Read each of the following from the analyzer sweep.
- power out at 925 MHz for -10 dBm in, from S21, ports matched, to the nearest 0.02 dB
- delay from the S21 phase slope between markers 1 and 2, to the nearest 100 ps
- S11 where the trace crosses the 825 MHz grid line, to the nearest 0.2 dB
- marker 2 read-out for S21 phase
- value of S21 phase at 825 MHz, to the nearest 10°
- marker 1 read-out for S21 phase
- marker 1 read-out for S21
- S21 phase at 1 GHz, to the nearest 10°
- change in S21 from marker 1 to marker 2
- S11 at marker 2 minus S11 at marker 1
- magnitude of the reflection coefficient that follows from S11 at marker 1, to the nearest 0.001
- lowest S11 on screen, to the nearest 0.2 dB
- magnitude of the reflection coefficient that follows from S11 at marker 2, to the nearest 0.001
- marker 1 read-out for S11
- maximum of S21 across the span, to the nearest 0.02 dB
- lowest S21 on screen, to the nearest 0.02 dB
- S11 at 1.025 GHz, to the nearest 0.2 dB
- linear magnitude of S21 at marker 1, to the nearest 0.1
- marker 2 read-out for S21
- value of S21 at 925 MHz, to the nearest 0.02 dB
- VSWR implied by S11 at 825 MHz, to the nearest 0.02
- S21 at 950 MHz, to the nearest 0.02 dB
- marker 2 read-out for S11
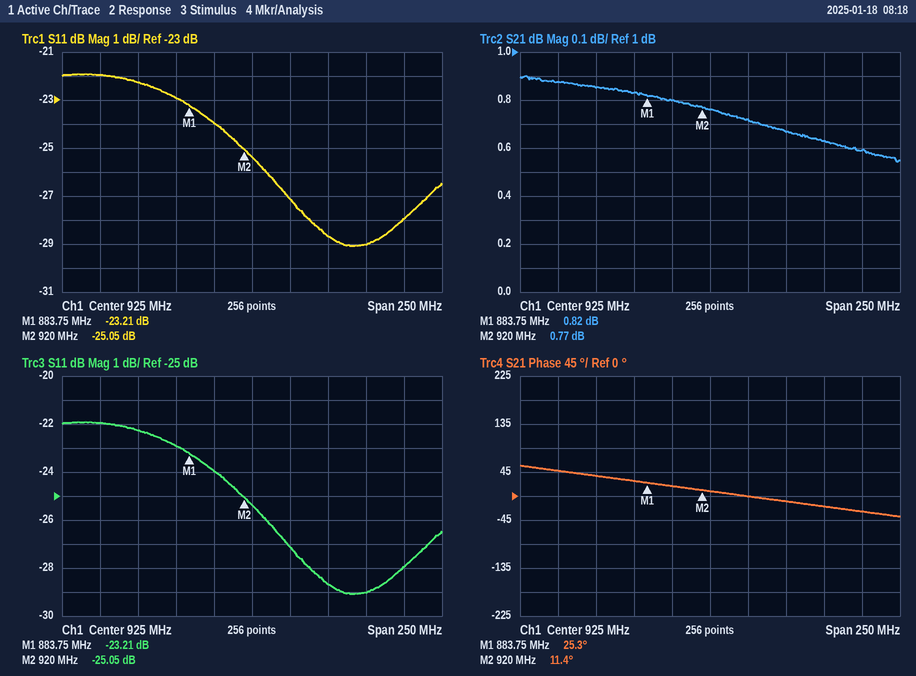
-9.24 dBm
1.1 ns
-22.0 dB
11.4°
50°
25.3°
0.82 dB
-20°
-0.05 dB
-1.84 dB
0.069
-29.0 dB
0.056
-23.21 dB
0.90 dB
0.54 dB
-28.0 dB
1.1
0.77 dB
0.76 dB
1.18
0.72 dB
-25.05 dB
